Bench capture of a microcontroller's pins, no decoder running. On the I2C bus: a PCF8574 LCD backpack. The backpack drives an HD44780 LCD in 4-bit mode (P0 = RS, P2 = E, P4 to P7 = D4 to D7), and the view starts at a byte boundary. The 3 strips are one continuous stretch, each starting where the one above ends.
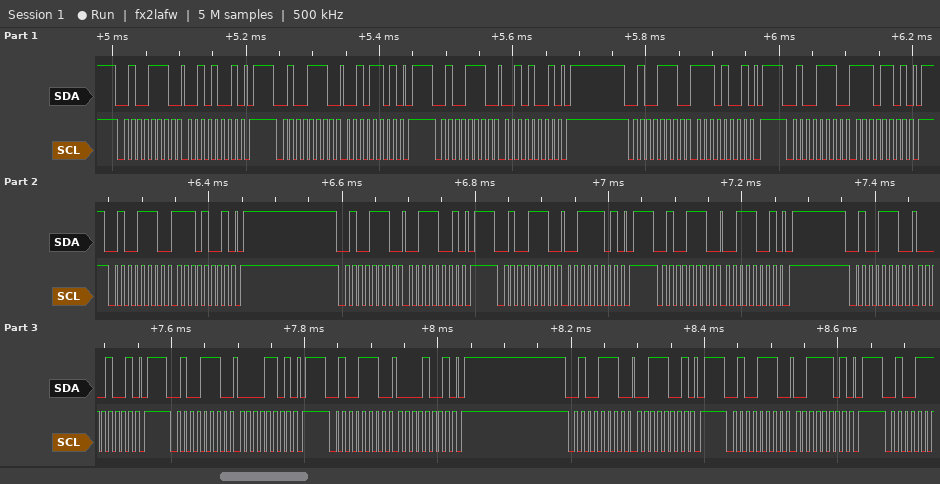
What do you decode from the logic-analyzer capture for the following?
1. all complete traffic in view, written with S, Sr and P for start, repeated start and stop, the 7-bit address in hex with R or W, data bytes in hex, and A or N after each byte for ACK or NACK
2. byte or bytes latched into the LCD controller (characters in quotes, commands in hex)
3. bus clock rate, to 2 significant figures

S 27W A 29 A P S 27W A 2D A P S 27W A 29 A P S 27W A E9 A P S 27W A ED A P S 27W A E9 A P S 27W A 39 A P S 27W A 3D A P S 27W A 39 A P S 27W A 09 A P S 27W A 0D A P S 27W A 09 A P S 27W A 39 A P S 27W A 3D A P
'.' '0'
100 kHz
